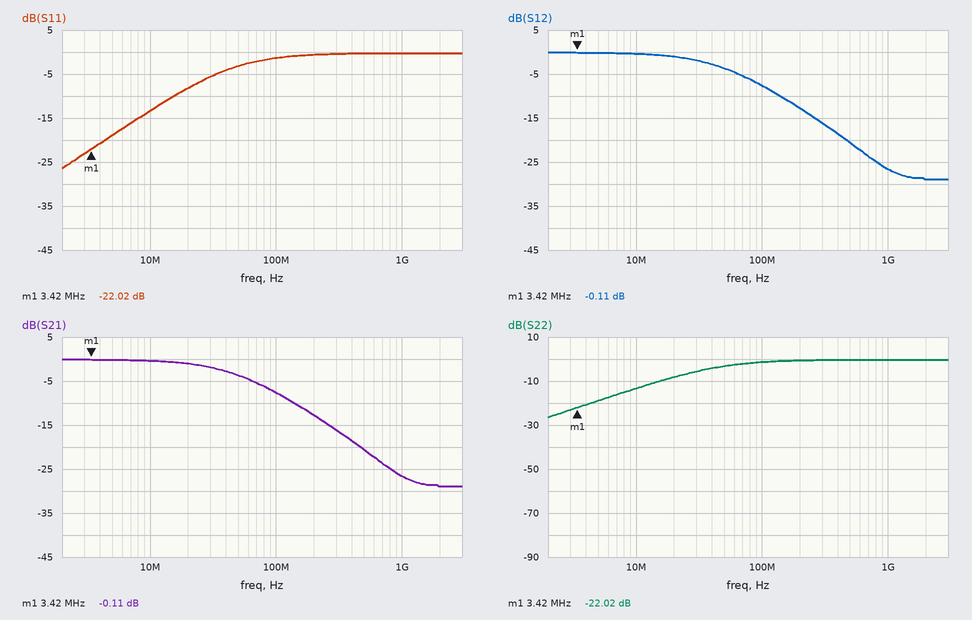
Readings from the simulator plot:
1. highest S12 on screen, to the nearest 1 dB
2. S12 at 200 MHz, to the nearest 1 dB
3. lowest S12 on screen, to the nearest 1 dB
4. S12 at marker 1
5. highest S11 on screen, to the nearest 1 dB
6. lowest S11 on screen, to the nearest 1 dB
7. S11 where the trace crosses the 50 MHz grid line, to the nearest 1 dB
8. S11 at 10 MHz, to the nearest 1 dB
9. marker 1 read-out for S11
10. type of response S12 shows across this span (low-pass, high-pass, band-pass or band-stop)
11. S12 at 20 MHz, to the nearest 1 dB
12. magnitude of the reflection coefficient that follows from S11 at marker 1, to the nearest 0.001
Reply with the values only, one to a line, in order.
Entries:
0 dB
-13 dB
-29 dB
-0.11 dB
0 dB
-26 dB
-3 dB
-13 dB
-22.02 dB
low-pass
-1 dB
0.079
